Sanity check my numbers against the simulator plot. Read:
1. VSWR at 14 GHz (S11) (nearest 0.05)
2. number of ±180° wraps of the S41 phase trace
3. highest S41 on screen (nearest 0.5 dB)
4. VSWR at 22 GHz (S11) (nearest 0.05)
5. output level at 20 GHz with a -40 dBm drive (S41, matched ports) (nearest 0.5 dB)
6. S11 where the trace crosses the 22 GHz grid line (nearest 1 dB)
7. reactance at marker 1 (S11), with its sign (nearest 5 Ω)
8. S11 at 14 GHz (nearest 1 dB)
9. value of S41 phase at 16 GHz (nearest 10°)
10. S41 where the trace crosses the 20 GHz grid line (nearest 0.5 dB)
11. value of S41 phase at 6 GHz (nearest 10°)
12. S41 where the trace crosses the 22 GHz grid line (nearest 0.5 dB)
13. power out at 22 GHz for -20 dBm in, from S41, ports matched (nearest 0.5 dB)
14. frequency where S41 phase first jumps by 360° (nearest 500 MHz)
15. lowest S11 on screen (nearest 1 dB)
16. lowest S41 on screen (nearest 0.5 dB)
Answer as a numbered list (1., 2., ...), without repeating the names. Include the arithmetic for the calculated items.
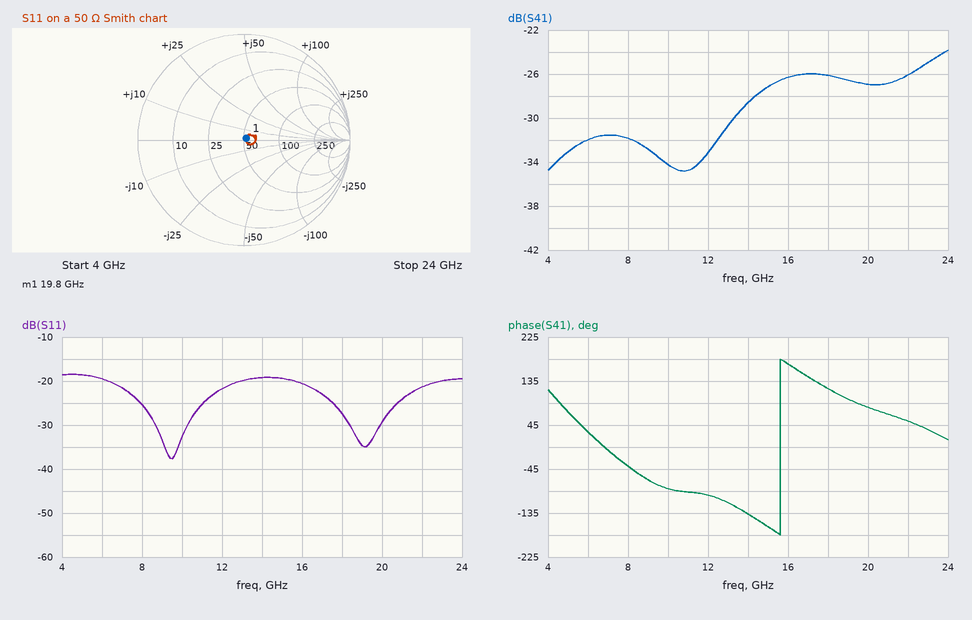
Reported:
1. |Γ| = 10^(-19/20) = 0.1122; VSWR = (1 + 0.1122)/(1 − 0.1122) ≈ 1.25
2. 1
3. -24.0 dB
4. |Γ| = 10^(-21/20) = 0.0891; VSWR = (1 + 0.0891)/(1 − 0.0891) ≈ 1.20
5. -40 dBm + (-27.0 dB) = -67.0 dBm
6. -21 dB
7. 0 Ω
8. -19 dB
9. 170°
10. -27.0 dB
11. 30°
12. -26.0 dB
13. -20 dBm + (-26.0 dB) = -46.0 dBm
14. 15.5 GHz
15. -38 dB
16. -35.0 dB
